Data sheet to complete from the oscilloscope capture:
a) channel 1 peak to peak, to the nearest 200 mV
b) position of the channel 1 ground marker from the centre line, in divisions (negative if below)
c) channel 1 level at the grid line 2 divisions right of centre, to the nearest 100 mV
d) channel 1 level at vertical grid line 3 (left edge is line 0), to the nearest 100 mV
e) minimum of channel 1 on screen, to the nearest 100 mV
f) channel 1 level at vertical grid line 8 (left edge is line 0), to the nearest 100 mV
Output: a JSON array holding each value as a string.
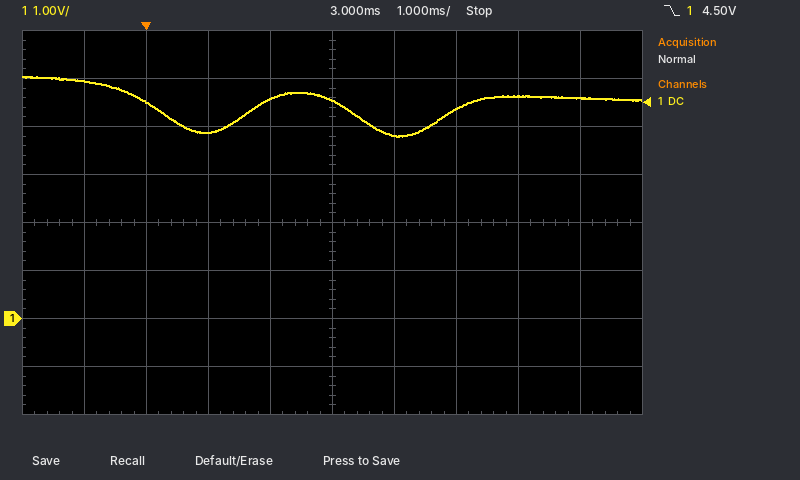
["1.2 V", "-2.0 div", "4.4 V", "3.9 V", "3.8 V", "4.6 V"]
